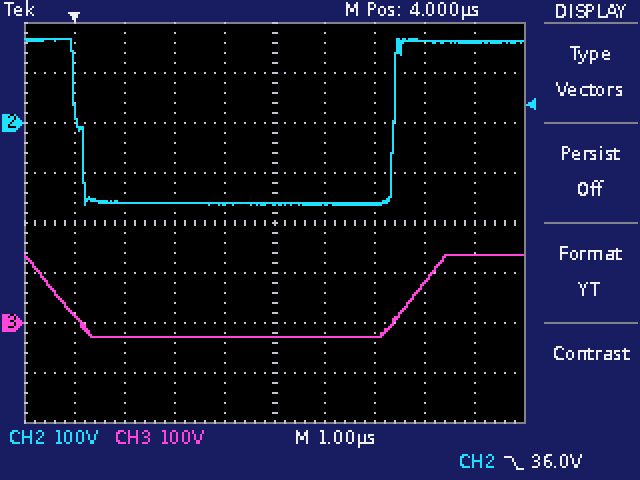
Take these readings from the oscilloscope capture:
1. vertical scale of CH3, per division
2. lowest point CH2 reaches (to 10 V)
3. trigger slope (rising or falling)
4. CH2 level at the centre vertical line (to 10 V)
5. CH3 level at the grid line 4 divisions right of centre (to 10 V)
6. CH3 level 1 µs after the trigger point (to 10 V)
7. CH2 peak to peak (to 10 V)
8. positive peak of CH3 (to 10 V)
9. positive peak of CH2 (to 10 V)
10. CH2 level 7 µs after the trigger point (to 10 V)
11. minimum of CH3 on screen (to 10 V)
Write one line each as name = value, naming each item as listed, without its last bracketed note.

vertical scale of CH3, per division = 100 V
lowest point CH2 reaches = -160 V
trigger slope = falling
CH2 level at the centre vertical line = -160 V
CH3 level at the grid line 4 divisions right of centre = 140 V
CH3 level 1 µs after the trigger point = -30 V
CH2 peak to peak = 330 V
positive peak of CH3 = 140 V
positive peak of CH2 = 170 V
CH2 level 7 µs after the trigger point = 160 V
minimum of CH3 on screen = -30 V
